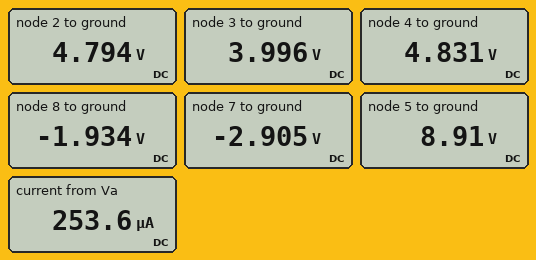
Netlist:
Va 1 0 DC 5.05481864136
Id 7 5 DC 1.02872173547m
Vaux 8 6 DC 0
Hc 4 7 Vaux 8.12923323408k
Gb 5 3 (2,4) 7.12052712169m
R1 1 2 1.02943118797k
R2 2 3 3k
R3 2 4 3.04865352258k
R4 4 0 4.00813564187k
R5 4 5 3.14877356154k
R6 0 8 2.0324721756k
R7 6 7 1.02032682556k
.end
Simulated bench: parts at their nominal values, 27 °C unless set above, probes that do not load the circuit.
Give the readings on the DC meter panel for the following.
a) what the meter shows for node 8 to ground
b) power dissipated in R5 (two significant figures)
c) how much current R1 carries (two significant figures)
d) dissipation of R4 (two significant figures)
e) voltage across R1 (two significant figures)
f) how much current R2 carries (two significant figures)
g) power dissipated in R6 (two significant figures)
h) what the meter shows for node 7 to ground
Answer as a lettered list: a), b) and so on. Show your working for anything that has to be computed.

a) -1.934 V
b) (8.91 V - 4.831 V)^2 / 3.149 kΩ = 5.3 mW
c) (5.055 V - 4.794 V) / 1.029 kΩ = 250 µA
d) (4.831 V)^2 / 4.008 kΩ = 5.8 mW
e) 5.055 V - 4.794 V = 260 mV
f) (4.794 V - 3.996 V) / 3 kΩ = 270 µA
g) (0 V - (-1.934 V))^2 / 2.032 kΩ = 1.8 mW
h) -2.905 V
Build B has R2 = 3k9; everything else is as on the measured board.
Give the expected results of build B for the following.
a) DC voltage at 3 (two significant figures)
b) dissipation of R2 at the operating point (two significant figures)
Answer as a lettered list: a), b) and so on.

a) 3.8 V
b) 280 µW
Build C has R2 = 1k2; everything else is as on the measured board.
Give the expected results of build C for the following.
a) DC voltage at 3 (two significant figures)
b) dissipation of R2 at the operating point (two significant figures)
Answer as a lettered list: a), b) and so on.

a) 4.5 V
b) 85 µW
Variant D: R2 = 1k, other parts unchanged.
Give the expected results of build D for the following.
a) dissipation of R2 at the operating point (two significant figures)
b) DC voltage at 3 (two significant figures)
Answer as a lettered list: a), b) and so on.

a) 71 µW
b) 4.5 V
